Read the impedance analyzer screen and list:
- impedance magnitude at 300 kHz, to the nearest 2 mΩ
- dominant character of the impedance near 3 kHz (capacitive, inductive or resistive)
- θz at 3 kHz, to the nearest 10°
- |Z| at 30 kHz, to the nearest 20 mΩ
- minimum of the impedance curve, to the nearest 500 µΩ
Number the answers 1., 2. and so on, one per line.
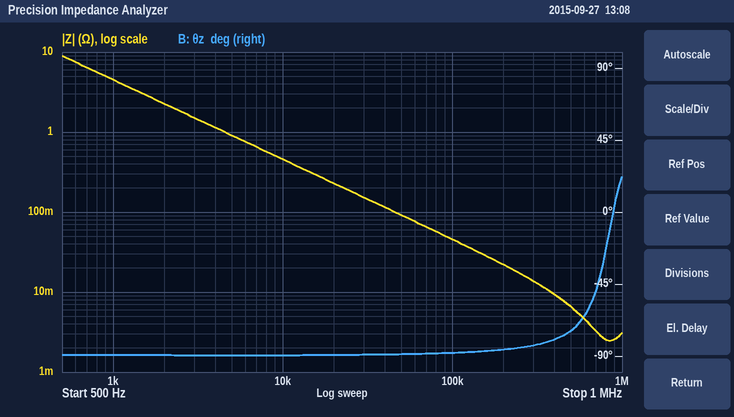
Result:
1. 14 mΩ
2. capacitive
3. -90°
4. 160 mΩ
5. 2.5 mΩ
